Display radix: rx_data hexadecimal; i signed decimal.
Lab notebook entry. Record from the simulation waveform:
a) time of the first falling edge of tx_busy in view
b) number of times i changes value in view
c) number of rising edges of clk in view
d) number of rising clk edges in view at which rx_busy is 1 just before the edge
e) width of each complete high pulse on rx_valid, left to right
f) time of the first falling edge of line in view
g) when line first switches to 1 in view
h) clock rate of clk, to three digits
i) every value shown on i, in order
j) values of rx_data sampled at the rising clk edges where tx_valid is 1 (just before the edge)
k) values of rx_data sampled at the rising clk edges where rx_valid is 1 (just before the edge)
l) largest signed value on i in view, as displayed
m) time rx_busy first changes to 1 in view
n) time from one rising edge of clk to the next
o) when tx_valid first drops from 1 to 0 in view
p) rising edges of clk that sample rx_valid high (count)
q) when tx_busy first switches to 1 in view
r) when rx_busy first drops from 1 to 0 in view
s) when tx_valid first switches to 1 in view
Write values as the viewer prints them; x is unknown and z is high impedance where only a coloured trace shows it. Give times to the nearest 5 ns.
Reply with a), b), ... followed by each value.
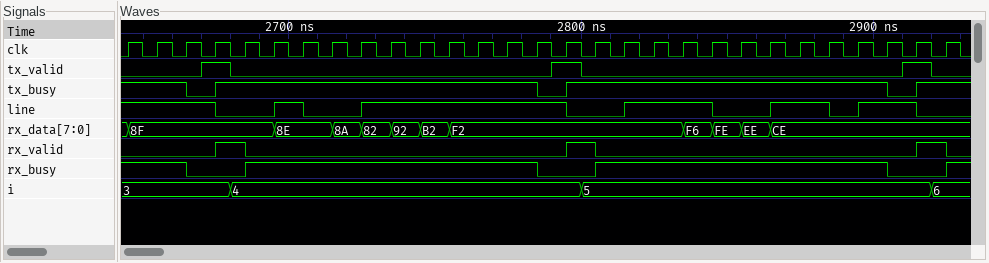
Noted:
a) 2665 ns
b) 3
c) 29
d) 23
e) 10 ns, 10 ns, 10 ns
f) 2675 ns
g) 2695 ns
h) 100 MHz
i) 3, 4, 5, 6
j) 8F, F2, CE
k) 8F, F2, CE
l) 6
m) 2685 ns
n) 10 ns
o) 2680 ns
p) 3
q) 2675 ns
r) 2665 ns
s) 2670 ns
